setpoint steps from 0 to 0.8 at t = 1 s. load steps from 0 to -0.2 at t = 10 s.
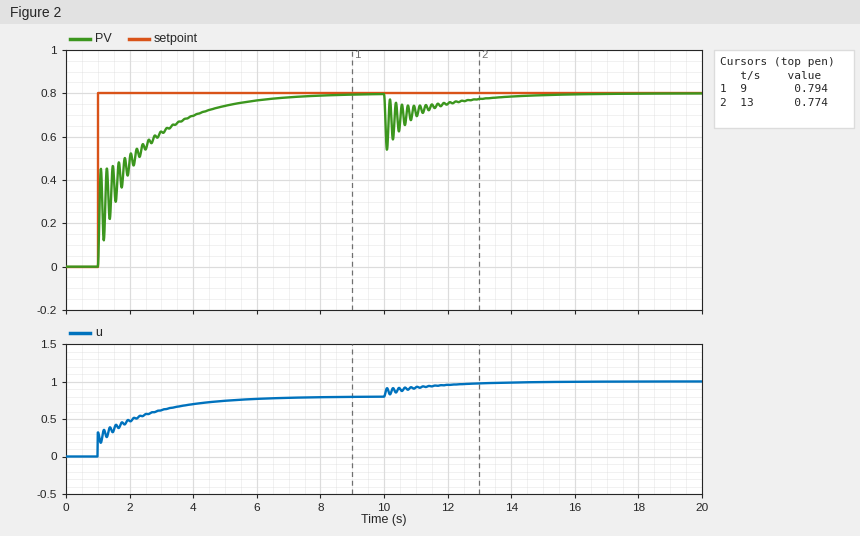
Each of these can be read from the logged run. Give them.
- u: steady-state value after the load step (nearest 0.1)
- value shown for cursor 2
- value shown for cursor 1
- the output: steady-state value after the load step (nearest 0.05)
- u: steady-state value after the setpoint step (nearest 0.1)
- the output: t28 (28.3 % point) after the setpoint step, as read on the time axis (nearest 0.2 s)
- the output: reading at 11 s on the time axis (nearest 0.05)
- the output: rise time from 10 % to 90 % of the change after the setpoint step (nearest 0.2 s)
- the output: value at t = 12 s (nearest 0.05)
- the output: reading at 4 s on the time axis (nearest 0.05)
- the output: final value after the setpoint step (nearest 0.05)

1.0
0.774
0.794
0.80
0.8
1.0 s
0.70
3.4 s
0.75
0.70
0.80
